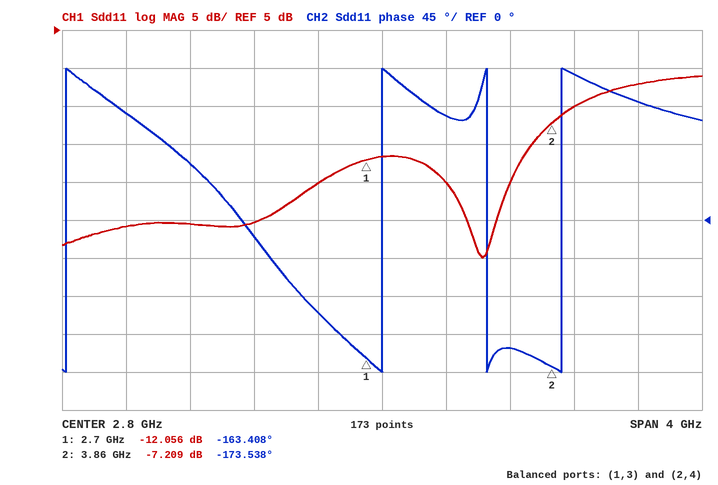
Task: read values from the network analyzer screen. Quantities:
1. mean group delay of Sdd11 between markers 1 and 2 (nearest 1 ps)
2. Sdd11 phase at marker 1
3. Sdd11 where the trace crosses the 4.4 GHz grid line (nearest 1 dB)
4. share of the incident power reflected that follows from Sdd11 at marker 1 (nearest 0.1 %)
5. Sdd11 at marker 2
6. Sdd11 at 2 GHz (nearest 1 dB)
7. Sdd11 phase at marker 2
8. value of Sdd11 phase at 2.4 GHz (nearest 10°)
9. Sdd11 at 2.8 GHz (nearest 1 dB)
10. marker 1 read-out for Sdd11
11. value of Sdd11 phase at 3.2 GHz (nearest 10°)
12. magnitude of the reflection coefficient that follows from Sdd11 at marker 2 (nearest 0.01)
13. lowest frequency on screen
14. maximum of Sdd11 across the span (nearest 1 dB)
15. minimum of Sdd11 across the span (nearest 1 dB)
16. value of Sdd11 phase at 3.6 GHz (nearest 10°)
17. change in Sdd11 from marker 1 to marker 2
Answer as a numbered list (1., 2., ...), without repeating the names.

1. 24 ps
2. -163.408°
3. -2 dB
4. 6.2 %
5. -7.209 dB
6. -20 dB
7. -173.538°
8. -110°
9. -12 dB
10. -12.056 dB
11. 120°
12. 0.44
13. 800 MHz
14. -1 dB
15. -25 dB
16. -150°
17. 4.847 dB
